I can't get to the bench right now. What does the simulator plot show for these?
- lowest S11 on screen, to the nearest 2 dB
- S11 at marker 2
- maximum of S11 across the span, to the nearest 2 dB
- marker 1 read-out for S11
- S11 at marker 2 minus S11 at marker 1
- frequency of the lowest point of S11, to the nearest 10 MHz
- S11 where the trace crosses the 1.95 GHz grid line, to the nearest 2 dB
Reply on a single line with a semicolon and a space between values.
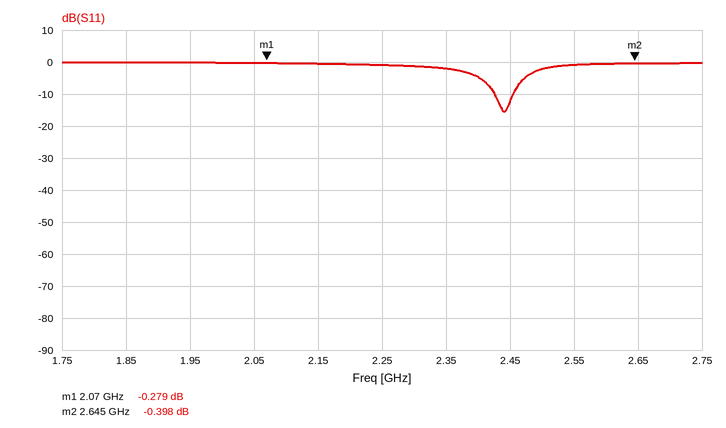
-16 dB; -0.398 dB; 0 dB; -0.279 dB; -0.119 dB; 2.44 GHz; 0 dB
